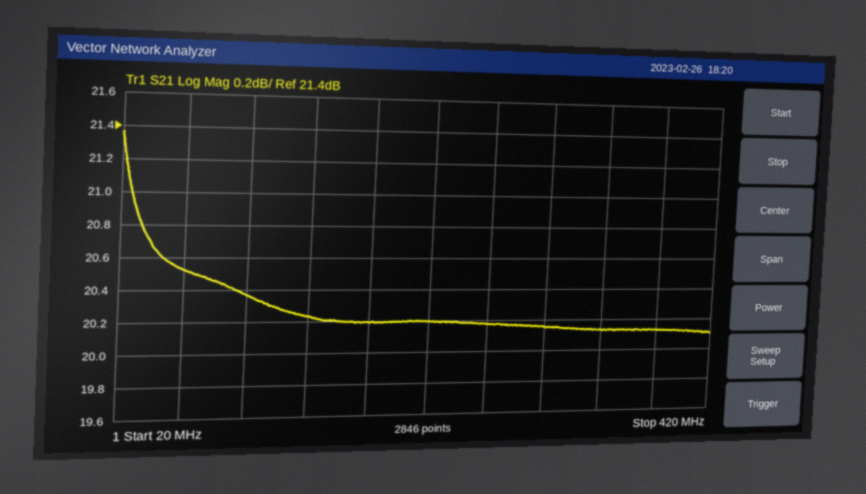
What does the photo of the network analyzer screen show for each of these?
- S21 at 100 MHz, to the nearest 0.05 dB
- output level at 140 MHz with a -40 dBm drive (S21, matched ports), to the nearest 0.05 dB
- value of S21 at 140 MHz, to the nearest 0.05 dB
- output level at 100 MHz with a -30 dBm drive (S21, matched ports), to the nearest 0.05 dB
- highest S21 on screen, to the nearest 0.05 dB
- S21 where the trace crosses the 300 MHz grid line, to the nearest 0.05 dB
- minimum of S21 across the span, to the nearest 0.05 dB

20.35 dB
-19.75 dBm
20.25 dB
-9.65 dBm
21.35 dB
20.15 dB
20.10 dB
